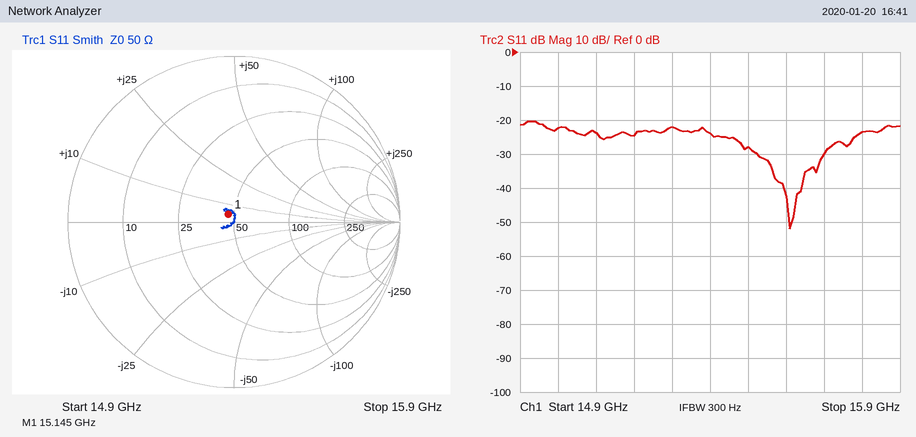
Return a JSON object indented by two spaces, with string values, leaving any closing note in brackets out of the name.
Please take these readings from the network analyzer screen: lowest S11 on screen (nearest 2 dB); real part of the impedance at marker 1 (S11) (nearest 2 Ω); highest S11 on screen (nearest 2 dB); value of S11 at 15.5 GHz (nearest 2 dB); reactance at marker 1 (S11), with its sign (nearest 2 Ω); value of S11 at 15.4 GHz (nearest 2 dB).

{
  "lowest S11 on screen": "-52 dB",
  "real part of the impedance at marker 1 (S11)": "46 Ω",
  "highest S11 on screen": "-20 dB",
  "value of S11 at 15.5 GHz": "-28 dB",
  "reactance at marker 1 (S11), with its sign": "+4 Ω",
  "value of S11 at 15.4 GHz": "-24 dB"
}
